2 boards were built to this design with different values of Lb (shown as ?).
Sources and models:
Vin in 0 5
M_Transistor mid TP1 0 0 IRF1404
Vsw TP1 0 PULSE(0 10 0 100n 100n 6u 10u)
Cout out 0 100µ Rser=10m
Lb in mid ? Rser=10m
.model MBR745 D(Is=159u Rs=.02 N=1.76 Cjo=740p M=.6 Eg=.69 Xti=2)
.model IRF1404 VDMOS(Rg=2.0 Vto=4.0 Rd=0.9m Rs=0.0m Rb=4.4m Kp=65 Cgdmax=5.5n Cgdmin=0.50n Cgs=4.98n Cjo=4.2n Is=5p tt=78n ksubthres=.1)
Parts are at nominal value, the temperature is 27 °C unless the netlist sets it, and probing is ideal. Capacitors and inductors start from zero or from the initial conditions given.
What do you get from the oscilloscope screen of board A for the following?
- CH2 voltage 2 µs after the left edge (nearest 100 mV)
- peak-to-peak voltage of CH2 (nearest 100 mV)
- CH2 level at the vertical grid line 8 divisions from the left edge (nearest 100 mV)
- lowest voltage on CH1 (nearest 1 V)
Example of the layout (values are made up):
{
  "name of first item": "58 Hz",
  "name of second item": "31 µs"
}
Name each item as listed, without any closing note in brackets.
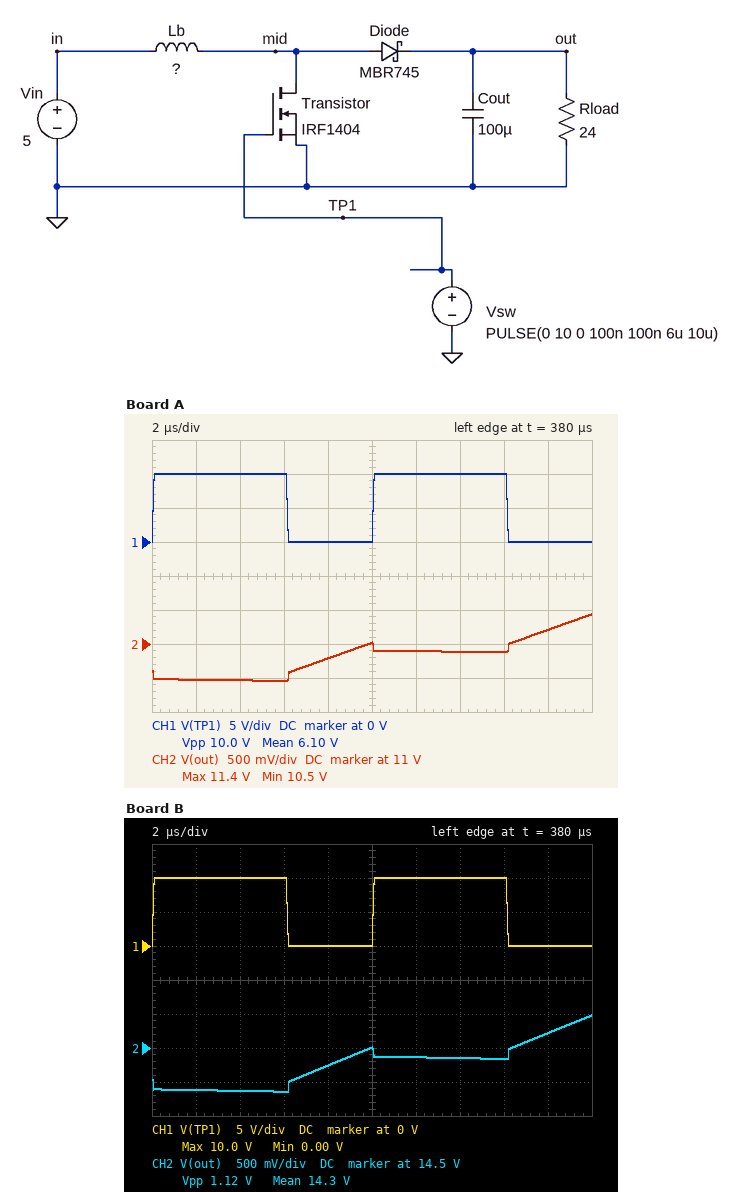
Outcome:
{
  "CH2 voltage 2 µs after the left edge": "10.5 V",
  "peak-to-peak voltage of CH2": "1.0 V",
  "CH2 level at the vertical grid line 8 divisions from the left edge": "10.9 V",
  "lowest voltage on CH1": "0 V"
}
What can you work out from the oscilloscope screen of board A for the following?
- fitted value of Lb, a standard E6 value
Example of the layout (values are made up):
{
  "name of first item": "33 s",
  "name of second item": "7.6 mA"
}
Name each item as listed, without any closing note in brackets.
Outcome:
{
  "fitted value of Lb, a standard E6 value": "100 µH"
}
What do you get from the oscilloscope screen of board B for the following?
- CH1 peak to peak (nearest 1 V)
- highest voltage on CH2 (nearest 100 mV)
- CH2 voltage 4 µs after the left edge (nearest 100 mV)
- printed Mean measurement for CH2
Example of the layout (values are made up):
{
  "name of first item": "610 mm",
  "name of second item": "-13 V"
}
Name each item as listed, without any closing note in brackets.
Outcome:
{
  "CH1 peak to peak": "10 V",
  "highest voltage on CH2": "15.0 V",
  "CH2 voltage 4 µs after the left edge": "13.9 V",
  "printed Mean measurement for CH2": "14.3 V"
}
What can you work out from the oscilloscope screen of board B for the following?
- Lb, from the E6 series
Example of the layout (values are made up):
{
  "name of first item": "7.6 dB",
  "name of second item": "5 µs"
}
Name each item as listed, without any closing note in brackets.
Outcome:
{
  "Lb, from the E6 series": "68 µH"
}
